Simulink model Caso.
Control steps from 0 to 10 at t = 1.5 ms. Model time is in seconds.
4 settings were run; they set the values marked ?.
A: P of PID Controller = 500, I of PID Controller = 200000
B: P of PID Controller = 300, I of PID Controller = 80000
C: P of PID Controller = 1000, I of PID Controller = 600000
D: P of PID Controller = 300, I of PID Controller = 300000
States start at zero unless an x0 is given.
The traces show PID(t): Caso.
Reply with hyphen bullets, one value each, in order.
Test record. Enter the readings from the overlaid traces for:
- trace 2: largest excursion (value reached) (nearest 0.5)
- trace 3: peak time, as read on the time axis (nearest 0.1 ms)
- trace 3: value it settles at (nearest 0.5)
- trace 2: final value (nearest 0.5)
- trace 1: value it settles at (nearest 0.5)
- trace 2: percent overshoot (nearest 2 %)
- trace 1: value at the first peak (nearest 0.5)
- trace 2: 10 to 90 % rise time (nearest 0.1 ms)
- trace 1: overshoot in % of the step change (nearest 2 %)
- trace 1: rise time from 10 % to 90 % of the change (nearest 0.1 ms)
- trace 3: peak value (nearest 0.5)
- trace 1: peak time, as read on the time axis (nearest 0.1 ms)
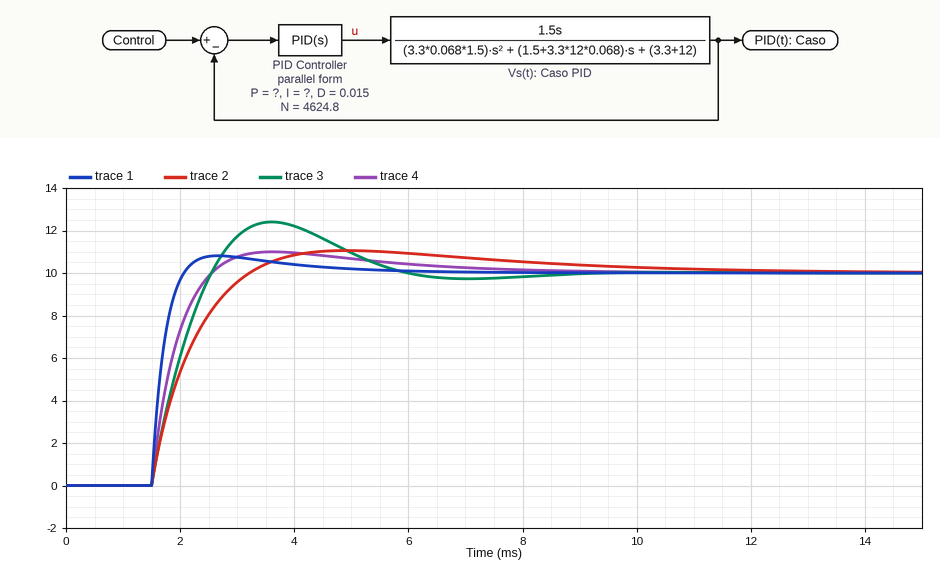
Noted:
- 11.0
- 3.6 ms
- 10.0
- 10.0
- 10.0
- 10 %
- 11.0
- 1.2 ms
- 8 %
- 0.4 ms
- 12.5
- 2.7 ms
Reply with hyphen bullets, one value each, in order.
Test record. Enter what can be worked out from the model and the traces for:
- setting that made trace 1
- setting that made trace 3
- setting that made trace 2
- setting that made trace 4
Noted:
- C
- D
- B
- A
